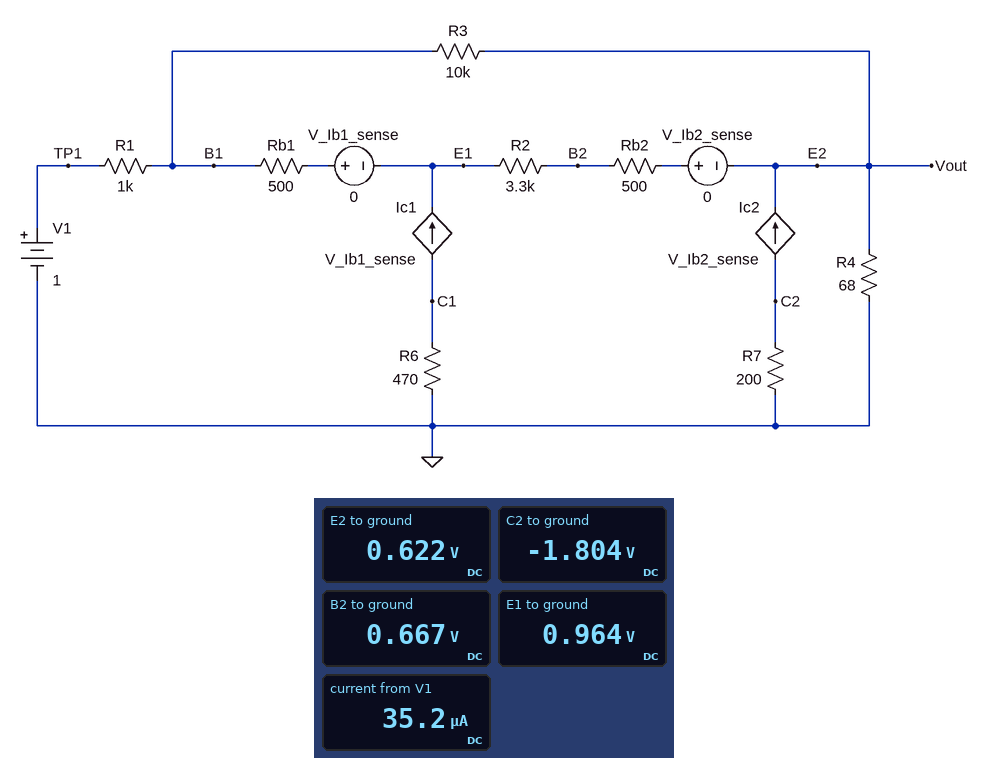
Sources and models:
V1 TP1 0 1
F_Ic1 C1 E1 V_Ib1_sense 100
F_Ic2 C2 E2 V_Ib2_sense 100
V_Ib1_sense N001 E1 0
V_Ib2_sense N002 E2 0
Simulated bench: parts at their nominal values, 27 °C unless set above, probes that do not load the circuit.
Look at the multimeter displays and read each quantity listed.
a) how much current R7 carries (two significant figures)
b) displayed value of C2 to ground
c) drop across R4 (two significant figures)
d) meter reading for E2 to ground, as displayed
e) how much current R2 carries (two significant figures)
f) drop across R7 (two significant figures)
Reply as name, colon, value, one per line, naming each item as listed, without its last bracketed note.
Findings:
how much current R7 carries: 9.0 mA
displayed value of C2 to ground: -1.804 V
drop across R4: 620 mV
meter reading for E2 to ground, as displayed: 0.622 V
how much current R2 carries: 90 µA
drop across R7: 1.8 V
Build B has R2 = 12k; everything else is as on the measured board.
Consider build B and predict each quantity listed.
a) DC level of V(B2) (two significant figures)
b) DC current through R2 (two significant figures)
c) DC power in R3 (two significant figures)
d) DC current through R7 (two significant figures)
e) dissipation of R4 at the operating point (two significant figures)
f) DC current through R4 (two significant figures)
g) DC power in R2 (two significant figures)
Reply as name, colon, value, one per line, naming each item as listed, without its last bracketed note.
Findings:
DC level of V(B2): 360 mV
DC current through R2: 48 µA
DC power in R3: 36 µW
DC current through R7: 4.8 mA
dissipation of R4 at the operating point: 1.7 mW
DC current through R4: 4.9 mA
DC power in R2: 28 µW
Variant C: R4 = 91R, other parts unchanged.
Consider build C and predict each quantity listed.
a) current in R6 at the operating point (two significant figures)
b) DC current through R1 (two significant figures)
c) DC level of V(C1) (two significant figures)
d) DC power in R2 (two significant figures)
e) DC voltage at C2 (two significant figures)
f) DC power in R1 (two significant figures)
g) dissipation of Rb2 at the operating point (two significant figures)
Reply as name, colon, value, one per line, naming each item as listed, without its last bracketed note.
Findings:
current in R6 at the operating point: 74 µA
DC current through R1: 29 µA
DC level of V(C1): -35 mV
DC power in R2: 18 µW
DC voltage at C2: -1.5 V
DC power in R1: 850 nW
dissipation of Rb2 at the operating point: 2.8 µW
